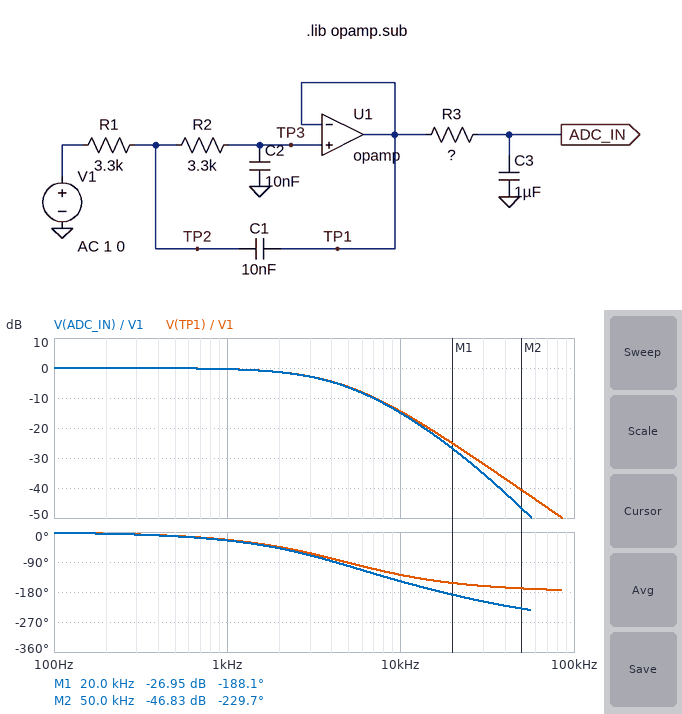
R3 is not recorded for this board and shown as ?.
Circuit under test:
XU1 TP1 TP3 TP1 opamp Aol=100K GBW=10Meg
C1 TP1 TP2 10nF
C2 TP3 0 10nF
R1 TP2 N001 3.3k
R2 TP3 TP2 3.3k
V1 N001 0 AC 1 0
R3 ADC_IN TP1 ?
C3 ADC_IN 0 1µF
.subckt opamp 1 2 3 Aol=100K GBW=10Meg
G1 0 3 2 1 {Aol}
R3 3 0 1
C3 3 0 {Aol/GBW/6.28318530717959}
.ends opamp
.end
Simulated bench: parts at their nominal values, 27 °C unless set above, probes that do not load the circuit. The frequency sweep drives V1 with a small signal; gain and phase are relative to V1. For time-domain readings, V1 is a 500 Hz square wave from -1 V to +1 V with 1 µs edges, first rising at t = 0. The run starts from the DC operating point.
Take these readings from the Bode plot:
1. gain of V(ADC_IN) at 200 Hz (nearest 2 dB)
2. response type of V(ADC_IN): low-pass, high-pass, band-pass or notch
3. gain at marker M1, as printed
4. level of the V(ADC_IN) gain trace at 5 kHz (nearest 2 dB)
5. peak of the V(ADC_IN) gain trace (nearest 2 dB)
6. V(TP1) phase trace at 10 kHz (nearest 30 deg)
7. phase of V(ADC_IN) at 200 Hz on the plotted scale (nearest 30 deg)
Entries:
0 dB
low-pass
-26.95 dB
-6 dB
0 dB
-120 deg
0 deg
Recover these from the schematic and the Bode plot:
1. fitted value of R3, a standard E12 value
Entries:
5.6 Ω
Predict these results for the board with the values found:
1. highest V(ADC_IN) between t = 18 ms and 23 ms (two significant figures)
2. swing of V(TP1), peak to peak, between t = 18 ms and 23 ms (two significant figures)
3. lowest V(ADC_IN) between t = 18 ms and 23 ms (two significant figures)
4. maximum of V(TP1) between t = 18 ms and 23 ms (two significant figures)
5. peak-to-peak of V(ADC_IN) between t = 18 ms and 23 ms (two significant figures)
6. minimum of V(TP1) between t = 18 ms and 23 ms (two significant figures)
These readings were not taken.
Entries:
1.0 V
2.0 V
-1.0 V
1.0 V
2.0 V
-1.0 V
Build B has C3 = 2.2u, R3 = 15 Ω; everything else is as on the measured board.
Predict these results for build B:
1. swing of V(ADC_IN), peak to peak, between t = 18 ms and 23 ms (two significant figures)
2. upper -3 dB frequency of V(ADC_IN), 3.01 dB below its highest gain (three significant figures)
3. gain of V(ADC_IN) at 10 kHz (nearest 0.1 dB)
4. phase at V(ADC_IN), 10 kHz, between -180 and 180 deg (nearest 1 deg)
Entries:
2.0 V
2.46 kHz
-21.7 dB
167 deg
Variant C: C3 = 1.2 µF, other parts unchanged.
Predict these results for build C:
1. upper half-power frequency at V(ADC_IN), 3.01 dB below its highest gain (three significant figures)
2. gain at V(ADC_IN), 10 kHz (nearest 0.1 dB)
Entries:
3.06 kHz
-15.2 dB
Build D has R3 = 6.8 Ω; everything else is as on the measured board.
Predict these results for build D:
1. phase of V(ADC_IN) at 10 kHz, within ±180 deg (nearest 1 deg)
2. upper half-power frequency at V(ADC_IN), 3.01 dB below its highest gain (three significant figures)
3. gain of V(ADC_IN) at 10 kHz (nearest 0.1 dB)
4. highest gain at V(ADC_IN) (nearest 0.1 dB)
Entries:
-152 deg
3.06 kHz
-15.2 dB
0 dB
